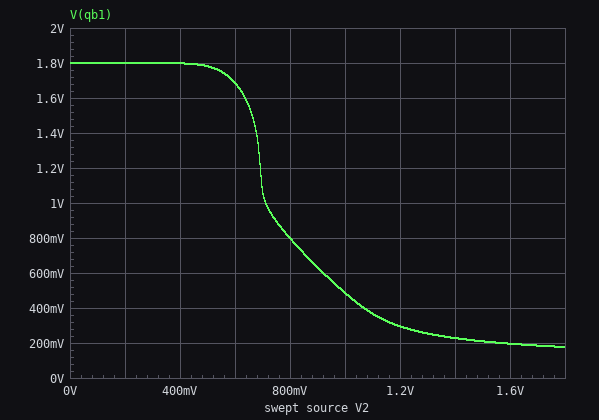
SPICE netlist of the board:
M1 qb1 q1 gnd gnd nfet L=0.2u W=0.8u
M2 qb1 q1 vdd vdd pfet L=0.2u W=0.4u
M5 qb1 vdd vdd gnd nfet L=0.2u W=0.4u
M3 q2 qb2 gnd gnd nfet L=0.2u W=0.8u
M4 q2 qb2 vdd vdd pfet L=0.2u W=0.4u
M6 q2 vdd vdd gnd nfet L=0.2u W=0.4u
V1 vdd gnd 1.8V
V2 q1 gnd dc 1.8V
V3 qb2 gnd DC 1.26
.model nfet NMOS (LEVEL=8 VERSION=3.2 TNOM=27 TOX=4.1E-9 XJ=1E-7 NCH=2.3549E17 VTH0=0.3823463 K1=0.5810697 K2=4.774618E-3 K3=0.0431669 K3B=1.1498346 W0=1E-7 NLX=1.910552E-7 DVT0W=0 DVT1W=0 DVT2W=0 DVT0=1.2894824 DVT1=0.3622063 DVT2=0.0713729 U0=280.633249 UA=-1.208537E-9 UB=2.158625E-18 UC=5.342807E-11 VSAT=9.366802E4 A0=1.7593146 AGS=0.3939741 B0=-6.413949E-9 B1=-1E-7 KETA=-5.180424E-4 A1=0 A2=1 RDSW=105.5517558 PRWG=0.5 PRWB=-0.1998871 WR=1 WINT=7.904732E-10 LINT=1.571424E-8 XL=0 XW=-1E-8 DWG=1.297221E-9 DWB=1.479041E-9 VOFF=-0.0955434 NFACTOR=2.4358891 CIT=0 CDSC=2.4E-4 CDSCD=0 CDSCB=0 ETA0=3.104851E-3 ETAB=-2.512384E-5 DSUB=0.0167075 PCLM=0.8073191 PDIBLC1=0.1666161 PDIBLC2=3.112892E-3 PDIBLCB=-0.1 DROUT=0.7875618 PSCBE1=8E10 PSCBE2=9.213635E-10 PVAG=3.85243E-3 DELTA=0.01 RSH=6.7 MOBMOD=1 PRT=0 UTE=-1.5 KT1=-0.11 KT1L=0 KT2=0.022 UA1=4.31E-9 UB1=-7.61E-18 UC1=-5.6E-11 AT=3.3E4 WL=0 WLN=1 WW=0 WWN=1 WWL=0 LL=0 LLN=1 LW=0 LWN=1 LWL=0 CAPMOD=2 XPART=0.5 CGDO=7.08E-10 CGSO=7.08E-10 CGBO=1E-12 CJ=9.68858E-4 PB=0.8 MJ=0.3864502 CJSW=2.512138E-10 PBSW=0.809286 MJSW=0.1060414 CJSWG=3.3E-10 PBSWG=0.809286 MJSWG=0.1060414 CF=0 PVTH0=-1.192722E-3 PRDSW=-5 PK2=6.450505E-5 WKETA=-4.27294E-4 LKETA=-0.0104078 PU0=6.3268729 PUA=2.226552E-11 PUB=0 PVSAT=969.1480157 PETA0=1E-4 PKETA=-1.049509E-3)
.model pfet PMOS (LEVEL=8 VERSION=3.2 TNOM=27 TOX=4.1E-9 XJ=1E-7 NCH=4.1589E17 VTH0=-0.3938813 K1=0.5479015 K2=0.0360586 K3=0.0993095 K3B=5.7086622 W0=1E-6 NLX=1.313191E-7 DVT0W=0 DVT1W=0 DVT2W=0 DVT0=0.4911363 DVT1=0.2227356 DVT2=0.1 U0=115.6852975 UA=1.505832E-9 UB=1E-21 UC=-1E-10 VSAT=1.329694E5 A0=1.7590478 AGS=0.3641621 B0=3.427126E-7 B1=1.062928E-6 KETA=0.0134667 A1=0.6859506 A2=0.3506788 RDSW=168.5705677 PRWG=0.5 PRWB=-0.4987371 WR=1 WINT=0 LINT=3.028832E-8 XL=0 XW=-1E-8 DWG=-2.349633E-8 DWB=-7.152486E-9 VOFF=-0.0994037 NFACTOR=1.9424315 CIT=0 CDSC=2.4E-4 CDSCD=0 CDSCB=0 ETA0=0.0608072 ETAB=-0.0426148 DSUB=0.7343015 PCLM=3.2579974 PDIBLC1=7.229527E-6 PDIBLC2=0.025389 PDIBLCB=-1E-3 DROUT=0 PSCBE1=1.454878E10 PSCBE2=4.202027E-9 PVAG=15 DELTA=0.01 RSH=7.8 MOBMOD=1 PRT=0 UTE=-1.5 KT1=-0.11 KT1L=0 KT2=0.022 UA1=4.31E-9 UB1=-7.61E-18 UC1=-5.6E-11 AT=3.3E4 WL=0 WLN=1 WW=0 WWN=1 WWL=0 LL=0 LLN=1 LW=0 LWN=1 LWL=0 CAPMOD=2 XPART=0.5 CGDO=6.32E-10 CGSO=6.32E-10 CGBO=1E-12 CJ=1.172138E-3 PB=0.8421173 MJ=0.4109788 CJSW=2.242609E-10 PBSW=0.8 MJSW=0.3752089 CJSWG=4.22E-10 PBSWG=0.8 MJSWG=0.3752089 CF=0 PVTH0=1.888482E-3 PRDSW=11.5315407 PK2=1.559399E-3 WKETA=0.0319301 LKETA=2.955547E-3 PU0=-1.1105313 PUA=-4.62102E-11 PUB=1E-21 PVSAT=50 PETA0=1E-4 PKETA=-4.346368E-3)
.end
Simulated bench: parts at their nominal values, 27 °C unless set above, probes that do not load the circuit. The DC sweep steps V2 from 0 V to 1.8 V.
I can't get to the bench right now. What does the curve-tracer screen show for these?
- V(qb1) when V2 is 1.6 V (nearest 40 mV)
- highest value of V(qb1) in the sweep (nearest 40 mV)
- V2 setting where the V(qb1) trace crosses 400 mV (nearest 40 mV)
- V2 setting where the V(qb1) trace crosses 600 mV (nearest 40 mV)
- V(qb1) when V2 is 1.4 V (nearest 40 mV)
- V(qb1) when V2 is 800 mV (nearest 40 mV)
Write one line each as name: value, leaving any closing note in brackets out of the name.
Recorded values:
V(qb1) when V2 is 1.6 V: 200 mV
highest value of V(qb1) in the sweep: 1.80 V
V2 setting where the V(qb1) trace crosses 400 mV: 1.08 V
V2 setting where the V(qb1) trace crosses 600 mV: 920 mV
V(qb1) when V2 is 1.4 V: 240 mV
V(qb1) when V2 is 800 mV: 800 mV
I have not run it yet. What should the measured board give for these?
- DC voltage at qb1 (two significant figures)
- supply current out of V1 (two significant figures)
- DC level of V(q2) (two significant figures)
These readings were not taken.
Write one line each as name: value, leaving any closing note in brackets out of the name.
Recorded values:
DC voltage at qb1: 180 mV
supply current out of V1: 340 µA
DC level of V(q2): 290 mV
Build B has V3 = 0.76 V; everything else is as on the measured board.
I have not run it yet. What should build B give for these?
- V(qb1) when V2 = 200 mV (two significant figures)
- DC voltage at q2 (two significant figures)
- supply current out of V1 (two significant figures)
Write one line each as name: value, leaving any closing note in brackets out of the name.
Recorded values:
V(qb1) when V2 = 200 mV: 1.8 V
DC voltage at q2: 890 mV
supply current out of V1: 220 µA
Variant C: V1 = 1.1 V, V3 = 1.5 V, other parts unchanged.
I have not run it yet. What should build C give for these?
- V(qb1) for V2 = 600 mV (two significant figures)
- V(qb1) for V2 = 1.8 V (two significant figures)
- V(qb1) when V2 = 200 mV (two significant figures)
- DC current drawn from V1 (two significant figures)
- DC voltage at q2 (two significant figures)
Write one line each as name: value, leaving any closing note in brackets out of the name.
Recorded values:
V(qb1) for V2 = 600 mV: 370 mV
V(qb1) for V2 = 1.8 V: 56 mV
V(qb1) when V2 = 200 mV: 1.1 V
DC current drawn from V1: 130 µA
DC voltage at q2: 71 mV
